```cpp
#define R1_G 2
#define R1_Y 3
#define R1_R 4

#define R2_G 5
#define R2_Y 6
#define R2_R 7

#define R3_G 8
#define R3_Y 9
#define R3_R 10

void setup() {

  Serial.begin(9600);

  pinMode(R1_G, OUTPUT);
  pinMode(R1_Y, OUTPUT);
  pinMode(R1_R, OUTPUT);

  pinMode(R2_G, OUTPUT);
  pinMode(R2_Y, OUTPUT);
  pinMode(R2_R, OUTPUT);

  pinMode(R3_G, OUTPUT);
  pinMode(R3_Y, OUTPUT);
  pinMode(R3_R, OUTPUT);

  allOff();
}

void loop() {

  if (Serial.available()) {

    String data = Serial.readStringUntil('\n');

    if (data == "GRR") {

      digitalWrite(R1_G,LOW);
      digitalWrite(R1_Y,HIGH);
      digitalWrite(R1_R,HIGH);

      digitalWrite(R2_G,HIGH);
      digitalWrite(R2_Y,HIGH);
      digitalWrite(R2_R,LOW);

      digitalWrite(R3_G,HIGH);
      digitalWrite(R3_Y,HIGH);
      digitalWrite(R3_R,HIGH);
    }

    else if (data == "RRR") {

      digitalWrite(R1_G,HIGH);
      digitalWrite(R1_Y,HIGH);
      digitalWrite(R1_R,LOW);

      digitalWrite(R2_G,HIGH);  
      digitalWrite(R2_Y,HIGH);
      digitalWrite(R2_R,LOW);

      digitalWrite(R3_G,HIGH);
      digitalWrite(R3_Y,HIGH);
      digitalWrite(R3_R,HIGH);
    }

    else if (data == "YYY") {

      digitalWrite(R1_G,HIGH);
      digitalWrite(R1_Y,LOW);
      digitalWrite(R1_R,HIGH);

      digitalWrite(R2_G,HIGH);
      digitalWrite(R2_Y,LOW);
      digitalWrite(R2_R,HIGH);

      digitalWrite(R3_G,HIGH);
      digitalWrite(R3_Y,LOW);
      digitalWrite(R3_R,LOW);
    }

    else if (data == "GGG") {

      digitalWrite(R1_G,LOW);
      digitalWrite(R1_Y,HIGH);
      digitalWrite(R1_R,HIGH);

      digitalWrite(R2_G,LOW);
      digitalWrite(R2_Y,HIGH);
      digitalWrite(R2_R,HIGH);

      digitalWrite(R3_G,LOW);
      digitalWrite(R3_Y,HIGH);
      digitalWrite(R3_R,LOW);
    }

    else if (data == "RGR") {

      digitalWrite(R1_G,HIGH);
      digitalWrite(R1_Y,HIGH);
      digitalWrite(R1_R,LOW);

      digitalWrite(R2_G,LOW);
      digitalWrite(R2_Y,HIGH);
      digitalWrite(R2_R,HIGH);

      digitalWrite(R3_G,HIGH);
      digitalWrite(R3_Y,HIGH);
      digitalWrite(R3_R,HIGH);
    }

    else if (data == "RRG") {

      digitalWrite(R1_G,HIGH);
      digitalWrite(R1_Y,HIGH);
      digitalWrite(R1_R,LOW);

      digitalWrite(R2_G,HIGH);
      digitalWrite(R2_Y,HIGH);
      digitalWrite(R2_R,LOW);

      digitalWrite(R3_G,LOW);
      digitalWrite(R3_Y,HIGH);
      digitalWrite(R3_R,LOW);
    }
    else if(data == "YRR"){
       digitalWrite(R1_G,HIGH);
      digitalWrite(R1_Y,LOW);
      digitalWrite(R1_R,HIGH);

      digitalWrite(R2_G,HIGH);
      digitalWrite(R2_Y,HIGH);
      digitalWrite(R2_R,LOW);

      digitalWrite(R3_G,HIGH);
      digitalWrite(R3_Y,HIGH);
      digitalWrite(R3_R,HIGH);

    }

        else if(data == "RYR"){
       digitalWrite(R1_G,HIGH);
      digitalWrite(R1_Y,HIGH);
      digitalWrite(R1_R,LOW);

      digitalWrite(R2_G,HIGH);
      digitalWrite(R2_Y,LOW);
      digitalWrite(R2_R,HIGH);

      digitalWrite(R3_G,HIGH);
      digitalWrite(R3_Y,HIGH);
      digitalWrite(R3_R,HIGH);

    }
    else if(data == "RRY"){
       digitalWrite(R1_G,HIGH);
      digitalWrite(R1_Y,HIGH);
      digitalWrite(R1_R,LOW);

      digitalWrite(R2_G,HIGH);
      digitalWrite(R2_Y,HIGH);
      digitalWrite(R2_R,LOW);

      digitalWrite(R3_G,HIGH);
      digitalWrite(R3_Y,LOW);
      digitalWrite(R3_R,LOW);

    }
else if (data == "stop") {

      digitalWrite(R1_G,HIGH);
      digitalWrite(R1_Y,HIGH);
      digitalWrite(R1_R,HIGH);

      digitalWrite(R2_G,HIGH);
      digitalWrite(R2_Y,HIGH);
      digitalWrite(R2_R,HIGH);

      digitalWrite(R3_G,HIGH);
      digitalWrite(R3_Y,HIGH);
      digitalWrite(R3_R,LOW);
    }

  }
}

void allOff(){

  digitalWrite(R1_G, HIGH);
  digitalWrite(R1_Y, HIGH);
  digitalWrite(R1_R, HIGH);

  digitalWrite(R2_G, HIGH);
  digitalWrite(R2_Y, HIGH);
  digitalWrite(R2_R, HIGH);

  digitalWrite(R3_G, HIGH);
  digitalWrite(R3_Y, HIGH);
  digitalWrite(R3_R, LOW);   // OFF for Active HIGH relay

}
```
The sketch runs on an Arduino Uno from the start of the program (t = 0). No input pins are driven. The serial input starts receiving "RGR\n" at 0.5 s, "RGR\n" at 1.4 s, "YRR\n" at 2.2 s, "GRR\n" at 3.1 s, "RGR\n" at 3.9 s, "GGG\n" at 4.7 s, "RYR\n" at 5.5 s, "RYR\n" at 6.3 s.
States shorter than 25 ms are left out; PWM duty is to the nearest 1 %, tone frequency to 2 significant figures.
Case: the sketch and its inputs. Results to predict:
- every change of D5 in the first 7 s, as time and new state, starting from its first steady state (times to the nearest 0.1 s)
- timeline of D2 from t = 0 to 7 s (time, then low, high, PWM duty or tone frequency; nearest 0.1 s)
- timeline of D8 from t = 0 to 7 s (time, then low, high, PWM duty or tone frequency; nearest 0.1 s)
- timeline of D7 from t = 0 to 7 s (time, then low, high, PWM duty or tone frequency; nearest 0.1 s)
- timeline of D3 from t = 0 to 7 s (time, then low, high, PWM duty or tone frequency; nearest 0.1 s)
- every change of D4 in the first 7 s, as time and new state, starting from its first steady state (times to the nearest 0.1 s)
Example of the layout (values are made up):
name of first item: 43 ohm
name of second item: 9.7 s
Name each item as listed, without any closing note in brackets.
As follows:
every change of D5 in the first 7 s, as time and new state, starting from its first steady state: 0 s high; 0.5 s low; 2.2 s high; 3.9 s low; 5.5 s high
timeline of D2 from t = 0 to 7 s: 0 s high; 3.1 s low; 3.9 s high; 4.7 s low; 5.5 s high
timeline of D8 from t = 0 to 7 s: 0 s high; 4.7 s low; 5.5 s high
timeline of D7 from t = 0 to 7 s: 0 s high; 2.2 s low; 3.9 s high
timeline of D3 from t = 0 to 7 s: 0 s high; 2.2 s low; 3.1 s high
every change of D4 in the first 7 s, as time and new state, starting from its first steady state: 0 s high; 0.5 s low; 2.2 s high; 3.9 s low; 4.7 s high; 5.5 s low
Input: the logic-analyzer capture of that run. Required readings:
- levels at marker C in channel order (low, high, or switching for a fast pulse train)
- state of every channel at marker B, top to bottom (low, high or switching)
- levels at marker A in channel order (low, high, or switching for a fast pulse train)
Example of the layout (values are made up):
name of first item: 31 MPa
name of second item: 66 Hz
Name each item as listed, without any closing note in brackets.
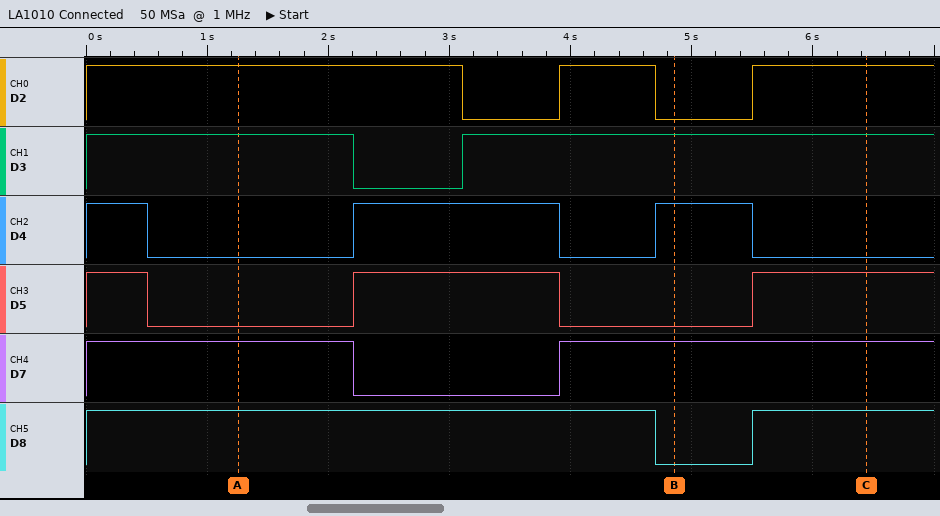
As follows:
levels at marker C in channel order: D2 high, D3 high, D4 low, D5 high, D7 high, D8 high
state of every channel at marker B, top to bottom: D2 low, D3 high, D4 high, D5 low, D7 high, D8 low
levels at marker A in channel order: D2 high, D3 high, D4 low, D5 low, D7 high, D8 high
